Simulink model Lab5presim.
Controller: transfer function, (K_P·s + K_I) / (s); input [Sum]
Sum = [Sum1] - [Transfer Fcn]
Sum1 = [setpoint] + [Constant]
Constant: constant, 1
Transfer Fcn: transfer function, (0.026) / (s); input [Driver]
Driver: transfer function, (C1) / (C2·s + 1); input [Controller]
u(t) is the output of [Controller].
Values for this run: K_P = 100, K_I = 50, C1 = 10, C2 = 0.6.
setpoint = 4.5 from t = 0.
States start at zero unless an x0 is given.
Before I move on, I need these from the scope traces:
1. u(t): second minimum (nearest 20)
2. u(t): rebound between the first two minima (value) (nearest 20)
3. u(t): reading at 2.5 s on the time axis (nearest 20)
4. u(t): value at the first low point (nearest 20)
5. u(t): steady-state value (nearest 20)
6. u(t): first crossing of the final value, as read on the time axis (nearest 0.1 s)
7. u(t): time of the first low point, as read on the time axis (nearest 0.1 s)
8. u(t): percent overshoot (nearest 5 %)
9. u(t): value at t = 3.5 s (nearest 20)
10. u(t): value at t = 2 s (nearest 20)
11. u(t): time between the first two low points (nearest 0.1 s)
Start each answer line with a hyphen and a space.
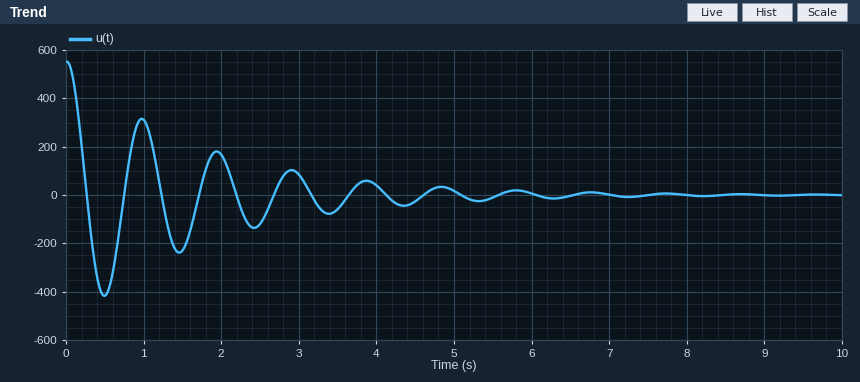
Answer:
- -240
- 320
- -120
- -420
- 0
- 0.3 s
- 0.5 s
- 75 %
- -60
- 160
- 1.0 s
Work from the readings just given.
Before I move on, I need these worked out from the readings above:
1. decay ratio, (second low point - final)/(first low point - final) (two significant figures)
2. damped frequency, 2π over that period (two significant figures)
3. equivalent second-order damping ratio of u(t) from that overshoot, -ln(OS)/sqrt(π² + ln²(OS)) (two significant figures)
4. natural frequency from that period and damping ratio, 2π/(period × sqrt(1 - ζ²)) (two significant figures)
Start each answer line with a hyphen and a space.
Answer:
- 0.57
- 6.3 rad/s
- 0.091
- 6.3 rad/s
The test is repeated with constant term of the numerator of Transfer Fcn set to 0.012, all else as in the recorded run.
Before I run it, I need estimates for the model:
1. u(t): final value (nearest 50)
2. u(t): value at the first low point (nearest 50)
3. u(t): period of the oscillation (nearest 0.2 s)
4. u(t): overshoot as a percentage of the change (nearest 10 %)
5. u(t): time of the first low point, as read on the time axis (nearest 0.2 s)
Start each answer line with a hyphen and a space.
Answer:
- 0
- -350
- 1.4 s
- 70 %
- 0.8 s
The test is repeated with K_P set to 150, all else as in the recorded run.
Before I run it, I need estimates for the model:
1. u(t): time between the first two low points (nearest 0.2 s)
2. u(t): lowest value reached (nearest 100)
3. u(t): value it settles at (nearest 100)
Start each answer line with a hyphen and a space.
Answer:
- 0.8 s
- -600
- 0
